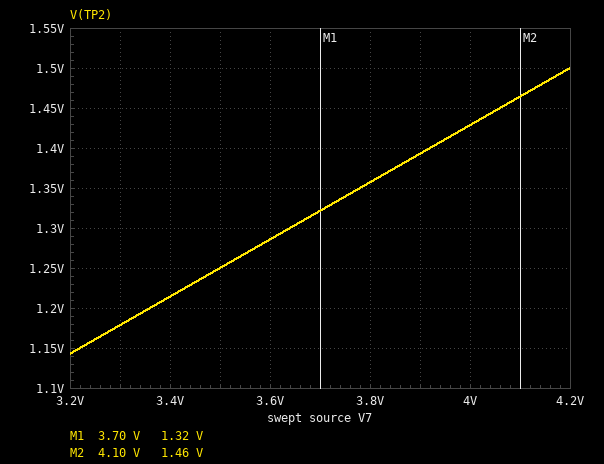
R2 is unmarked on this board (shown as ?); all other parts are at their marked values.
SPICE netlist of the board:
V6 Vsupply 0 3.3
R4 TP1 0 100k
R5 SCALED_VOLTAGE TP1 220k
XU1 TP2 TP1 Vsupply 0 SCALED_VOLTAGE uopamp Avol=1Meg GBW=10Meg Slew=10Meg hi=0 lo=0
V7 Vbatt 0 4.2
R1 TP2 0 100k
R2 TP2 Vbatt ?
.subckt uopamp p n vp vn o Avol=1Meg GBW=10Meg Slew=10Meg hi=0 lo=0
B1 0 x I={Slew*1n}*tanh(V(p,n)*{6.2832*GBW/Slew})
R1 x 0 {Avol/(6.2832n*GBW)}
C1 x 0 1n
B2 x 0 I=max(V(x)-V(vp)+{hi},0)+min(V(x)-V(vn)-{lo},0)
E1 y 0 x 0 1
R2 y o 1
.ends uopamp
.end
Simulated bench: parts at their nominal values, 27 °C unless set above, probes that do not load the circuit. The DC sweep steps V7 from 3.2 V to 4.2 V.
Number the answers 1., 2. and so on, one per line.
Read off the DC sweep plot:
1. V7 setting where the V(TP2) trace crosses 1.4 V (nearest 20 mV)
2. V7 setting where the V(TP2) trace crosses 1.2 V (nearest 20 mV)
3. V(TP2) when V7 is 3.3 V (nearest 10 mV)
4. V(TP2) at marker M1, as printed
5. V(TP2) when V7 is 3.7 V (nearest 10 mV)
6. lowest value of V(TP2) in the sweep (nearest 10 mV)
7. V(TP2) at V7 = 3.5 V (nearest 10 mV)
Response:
1. 3.92 V
2. 3.36 V
3. 1.18 V
4. 1.32 V
5. 1.32 V
6. 1.14 V
7. 1.25 V
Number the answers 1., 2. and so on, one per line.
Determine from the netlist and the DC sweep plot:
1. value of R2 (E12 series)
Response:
1. 180 kΩ
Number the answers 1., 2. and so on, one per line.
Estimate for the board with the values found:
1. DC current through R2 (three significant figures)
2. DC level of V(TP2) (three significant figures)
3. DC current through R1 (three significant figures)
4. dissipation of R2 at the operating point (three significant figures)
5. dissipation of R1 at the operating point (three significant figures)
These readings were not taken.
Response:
1. 15.0 µA
2. 1.50 V
3. 15.0 µA
4. 40.5 µW
5. 22.5 µW
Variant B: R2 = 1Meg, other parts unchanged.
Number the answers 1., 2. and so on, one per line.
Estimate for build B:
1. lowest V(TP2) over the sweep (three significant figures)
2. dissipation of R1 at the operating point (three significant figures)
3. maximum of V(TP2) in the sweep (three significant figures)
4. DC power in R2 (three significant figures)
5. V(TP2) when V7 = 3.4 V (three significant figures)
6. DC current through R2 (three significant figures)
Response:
1. 291 mV
2. 1.46 µW
3. 382 mV
4. 14.6 µW
5. 309 mV
6. 3.82 µA
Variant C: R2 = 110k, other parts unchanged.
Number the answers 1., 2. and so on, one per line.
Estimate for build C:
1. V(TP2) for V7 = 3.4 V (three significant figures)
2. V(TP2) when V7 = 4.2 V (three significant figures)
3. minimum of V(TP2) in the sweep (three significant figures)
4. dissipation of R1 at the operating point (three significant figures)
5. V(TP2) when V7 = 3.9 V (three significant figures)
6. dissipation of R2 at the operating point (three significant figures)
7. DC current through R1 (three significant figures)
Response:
1. 1.62 V
2. 2.00 V
3. 1.52 V
4. 40.0 µW
5. 1.86 V
6. 44.0 µW
7. 20.0 µA
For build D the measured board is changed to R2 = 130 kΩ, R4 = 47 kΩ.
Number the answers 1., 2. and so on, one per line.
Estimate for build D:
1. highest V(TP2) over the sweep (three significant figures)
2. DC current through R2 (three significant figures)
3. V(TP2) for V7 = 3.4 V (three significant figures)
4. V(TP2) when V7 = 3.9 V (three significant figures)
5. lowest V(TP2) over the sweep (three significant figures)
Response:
1. 1.83 V
2. 18.3 µA
3. 1.48 V
4. 1.70 V
5. 1.39 V
